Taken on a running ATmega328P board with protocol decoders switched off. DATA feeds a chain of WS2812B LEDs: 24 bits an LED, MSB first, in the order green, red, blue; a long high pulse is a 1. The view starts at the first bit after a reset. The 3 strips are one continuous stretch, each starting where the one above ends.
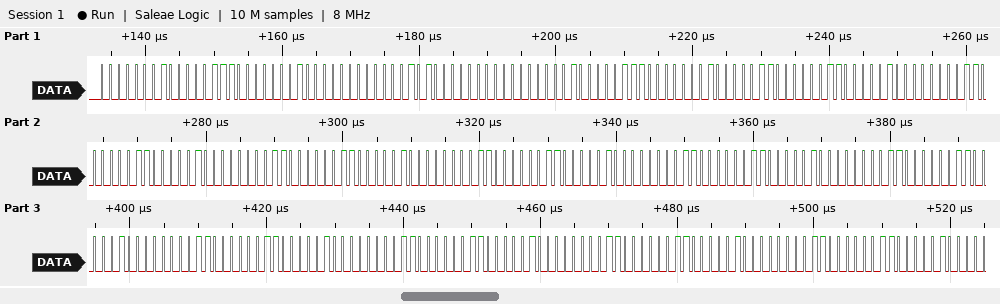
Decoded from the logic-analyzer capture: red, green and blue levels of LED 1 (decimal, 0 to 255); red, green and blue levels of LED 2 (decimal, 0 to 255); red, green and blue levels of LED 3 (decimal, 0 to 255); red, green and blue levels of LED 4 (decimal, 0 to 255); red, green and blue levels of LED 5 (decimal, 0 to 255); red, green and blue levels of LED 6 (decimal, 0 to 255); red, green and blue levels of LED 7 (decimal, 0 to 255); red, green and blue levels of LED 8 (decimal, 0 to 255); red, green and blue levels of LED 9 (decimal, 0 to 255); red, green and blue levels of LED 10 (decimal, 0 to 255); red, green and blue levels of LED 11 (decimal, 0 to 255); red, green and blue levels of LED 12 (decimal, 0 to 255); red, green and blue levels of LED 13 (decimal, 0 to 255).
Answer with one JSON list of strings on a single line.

["7, 1, 1", "10, 0, 0", "7, 1, 1", "6, 6, 8", "6, 6, 8", "6, 6, 8", "6, 6, 8", "6, 6, 8", "6, 6, 8", "6, 6, 8", "6, 6, 8", "6, 6, 8", "6, 6, 8"]
